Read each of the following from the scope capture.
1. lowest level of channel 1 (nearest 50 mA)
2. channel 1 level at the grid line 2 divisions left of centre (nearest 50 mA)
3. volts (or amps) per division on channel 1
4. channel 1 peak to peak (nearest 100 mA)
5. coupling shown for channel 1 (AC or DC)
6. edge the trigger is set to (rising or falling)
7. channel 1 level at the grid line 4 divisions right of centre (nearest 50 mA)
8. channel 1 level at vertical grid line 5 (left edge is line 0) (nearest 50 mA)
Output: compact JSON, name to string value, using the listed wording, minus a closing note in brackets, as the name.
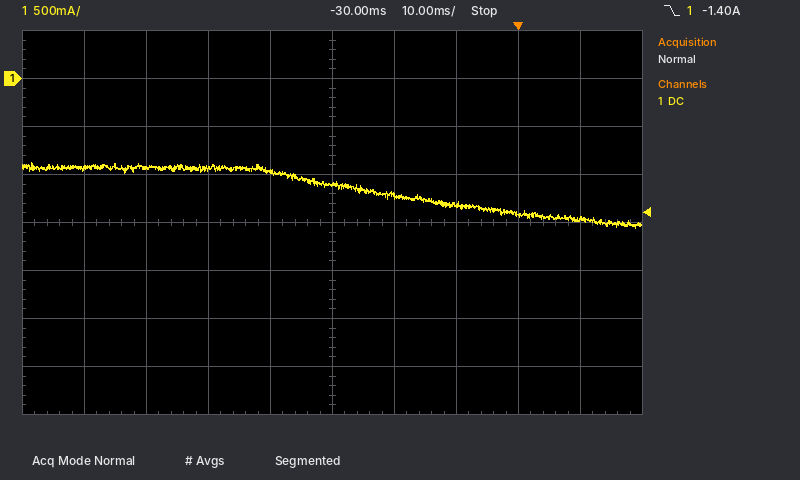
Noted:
{"lowest level of channel 1": "-1.55 A", "channel 1 level at the grid line 2 divisions left of centre": "-950 mA", "volts (or amps) per division on channel 1": "500 mA", "channel 1 peak to peak": "700 mA", "coupling shown for channel 1": "DC", "edge the trigger is set to": "falling", "channel 1 level at the grid line 4 divisions right of centre": "-1.45 A", "channel 1 level at vertical grid line 5 (left edge is line 0)": "-1.10 A"}
